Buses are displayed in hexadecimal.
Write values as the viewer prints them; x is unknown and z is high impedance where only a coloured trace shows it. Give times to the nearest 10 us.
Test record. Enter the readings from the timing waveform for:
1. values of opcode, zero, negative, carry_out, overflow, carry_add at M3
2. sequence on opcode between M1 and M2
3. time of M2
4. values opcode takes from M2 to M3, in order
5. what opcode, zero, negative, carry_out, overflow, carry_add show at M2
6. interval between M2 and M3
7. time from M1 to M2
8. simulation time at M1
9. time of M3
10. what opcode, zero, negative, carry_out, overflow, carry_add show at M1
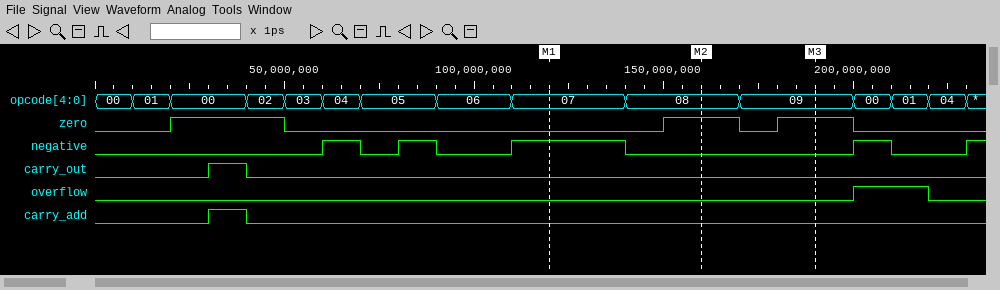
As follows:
opcode=09, zero=1, negative=0, carry_out=0, overflow=0, carry_add=0
07, 08
160 us
08, 09
opcode=08, zero=1, negative=0, carry_out=0, overflow=0, carry_add=0
30 us
40 us
120 us
190 us
opcode=07, zero=0, negative=1, carry_out=0, overflow=0, carry_add=0
